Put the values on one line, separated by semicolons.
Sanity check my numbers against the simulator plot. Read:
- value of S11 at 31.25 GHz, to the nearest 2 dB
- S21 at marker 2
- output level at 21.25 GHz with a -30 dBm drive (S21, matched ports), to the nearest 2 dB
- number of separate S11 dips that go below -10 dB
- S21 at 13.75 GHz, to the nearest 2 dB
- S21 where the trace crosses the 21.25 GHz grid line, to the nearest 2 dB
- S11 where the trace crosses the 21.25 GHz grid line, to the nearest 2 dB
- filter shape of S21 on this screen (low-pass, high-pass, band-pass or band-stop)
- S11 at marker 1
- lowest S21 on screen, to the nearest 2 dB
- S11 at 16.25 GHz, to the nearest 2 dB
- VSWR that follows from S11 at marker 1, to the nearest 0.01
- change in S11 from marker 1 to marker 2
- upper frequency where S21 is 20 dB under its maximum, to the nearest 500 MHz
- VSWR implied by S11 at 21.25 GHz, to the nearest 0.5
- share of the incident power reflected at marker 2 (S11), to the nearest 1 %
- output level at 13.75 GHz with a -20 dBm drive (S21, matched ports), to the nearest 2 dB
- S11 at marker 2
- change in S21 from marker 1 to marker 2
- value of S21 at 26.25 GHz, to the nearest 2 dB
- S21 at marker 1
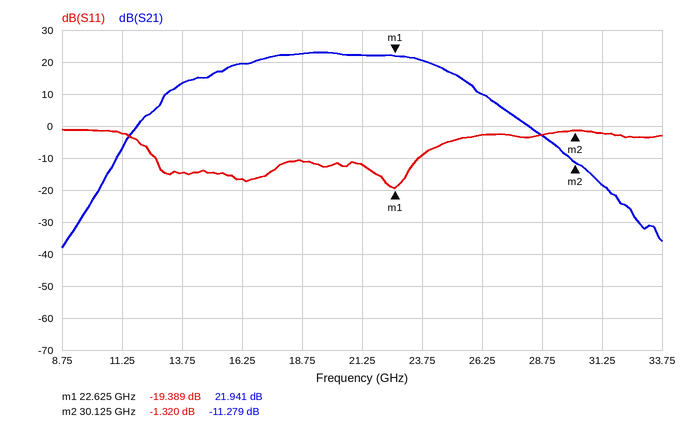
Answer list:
-2 dB; -11.279 dB; -8 dBm; 2; 14 dB; 22 dB; -12 dB; band-pass; -19.389 dB; -38 dB; -16 dB; 1.24; 18.069 dB; 27.5 GHz; 1.5; 74 %; -6 dBm; -1.320 dB; -33.220 dB; 10 dB; 21.941 dB
